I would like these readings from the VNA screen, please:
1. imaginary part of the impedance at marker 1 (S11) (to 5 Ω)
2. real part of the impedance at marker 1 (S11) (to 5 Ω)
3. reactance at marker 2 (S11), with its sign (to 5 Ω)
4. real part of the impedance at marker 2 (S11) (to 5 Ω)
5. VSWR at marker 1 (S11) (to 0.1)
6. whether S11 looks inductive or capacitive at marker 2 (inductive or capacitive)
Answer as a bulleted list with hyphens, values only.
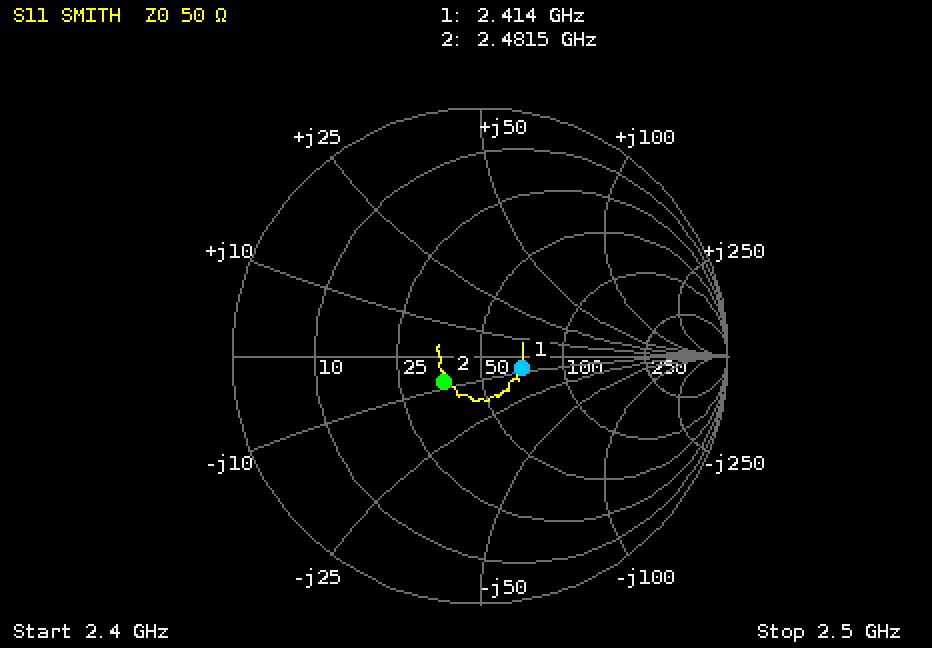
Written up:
- -5 Ω
- 70 Ω
- -10 Ω
- 35 Ω
- 1.4
- capacitive
